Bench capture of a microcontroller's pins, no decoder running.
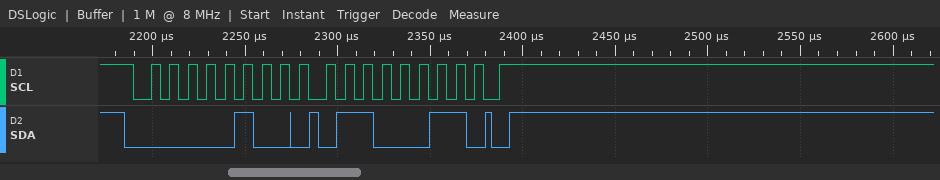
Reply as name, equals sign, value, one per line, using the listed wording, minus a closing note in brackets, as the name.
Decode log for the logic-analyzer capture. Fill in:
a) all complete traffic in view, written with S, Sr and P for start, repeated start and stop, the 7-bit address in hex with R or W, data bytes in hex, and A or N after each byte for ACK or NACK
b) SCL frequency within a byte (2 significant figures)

all complete traffic in view, written with S, Sr and P for start, repeated start and stop, the 7-bit address in hex with R or W, data bytes in hex, and A or N after each byte for ACK or NACK = S 02W A 63 A P
SCL frequency within a byte = 100 kHz
